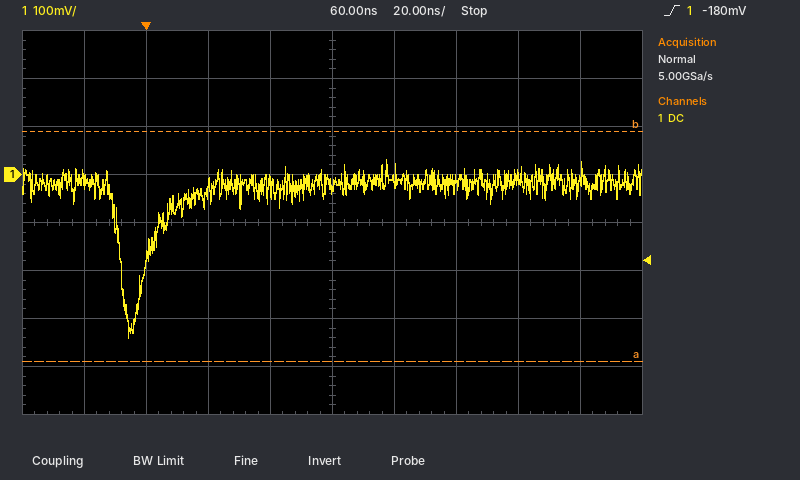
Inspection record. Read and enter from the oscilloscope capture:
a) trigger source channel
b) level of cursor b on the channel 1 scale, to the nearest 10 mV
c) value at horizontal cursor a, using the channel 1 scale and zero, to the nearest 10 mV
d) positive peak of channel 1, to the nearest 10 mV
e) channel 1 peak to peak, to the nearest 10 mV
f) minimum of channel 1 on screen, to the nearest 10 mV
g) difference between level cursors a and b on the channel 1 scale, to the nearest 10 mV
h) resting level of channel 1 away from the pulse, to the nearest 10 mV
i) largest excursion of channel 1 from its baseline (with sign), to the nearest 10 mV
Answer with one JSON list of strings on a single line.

["channel 1", "90 mV", "-390 mV", "30 mV", "370 mV", "-340 mV", "480 mV", "-20 mV", "-320 mV"]
